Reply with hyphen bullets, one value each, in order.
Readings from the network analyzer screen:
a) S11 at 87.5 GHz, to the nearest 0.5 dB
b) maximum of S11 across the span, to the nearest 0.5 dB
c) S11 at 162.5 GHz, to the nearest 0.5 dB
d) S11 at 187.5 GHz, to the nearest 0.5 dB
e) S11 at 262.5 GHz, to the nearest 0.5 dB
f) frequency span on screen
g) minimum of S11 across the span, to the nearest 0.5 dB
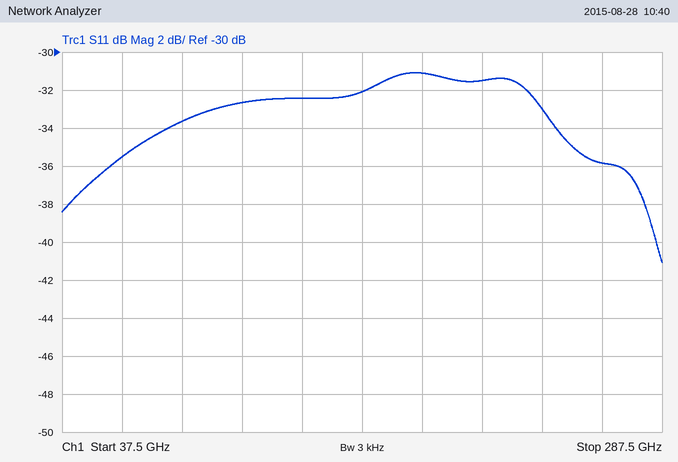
- -33.5 dB
- -31.0 dB
- -32.0 dB
- -31.0 dB
- -36.0 dB
- 250 GHz
- -41.0 dB
